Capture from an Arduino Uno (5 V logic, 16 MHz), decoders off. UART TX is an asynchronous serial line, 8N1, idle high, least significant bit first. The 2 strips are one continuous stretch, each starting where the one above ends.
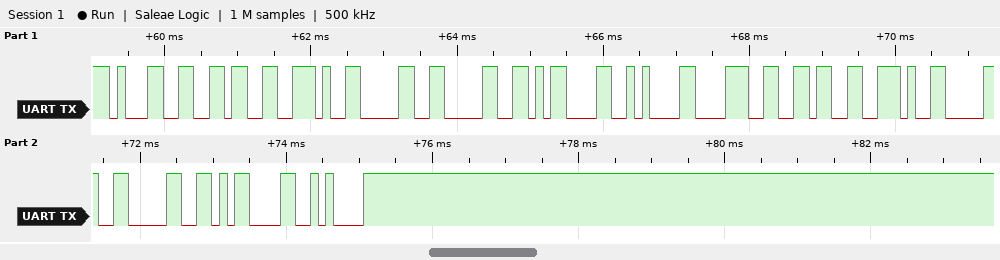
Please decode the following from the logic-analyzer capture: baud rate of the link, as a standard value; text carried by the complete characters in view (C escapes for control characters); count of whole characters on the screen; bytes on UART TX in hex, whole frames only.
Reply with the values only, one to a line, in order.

9600 baud
"16.00\r\n86.00\r\n"
14
0x31 0x36 0x2E 0x30 0x30 0x0D 0x0A 0x38 0x36 0x2E 0x30 0x30 0x0D 0x0A
